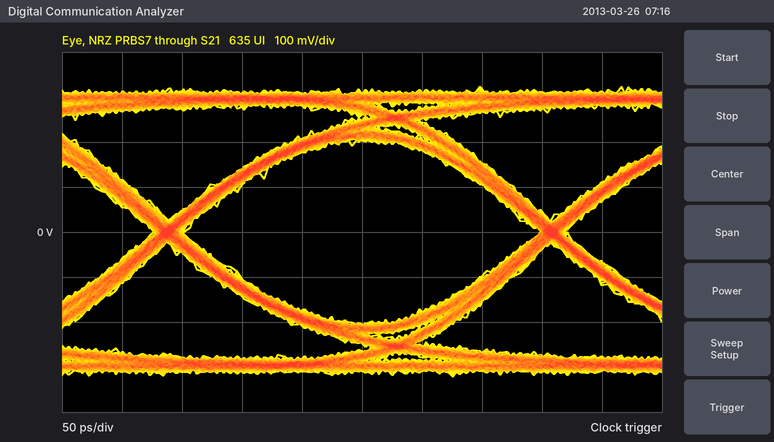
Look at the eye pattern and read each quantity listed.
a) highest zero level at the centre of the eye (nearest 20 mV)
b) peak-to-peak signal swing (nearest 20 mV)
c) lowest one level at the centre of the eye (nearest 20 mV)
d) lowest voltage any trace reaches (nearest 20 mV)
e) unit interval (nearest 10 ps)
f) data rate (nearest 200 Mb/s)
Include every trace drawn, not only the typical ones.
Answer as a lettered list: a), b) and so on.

a) -200 mV
b) 640 mV
c) 200 mV
d) -320 mV
e) 320 ps
f) 3.2 Gb/s
